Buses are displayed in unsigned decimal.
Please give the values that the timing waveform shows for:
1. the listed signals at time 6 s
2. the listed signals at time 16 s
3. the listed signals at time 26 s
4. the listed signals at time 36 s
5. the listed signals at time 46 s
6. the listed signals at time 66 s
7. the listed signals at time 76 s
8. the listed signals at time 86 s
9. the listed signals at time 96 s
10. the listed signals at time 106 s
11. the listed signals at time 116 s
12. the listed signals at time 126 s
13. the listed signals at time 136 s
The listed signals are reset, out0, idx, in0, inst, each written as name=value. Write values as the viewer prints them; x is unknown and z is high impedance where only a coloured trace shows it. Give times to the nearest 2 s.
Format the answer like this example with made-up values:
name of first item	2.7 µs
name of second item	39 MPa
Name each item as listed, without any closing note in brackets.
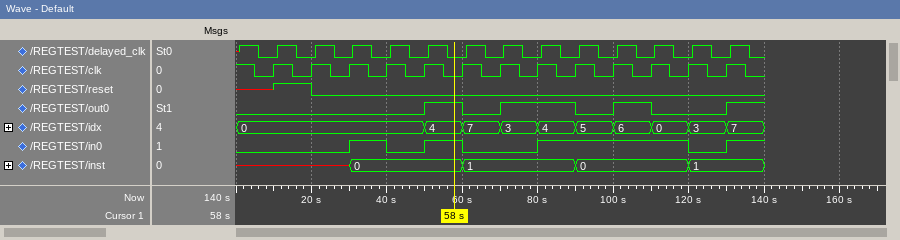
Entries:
the listed signals at time 6 s	reset=x, out0=0, idx=0, in0=0, inst=x
the listed signals at time 16 s	reset=1, out0=0, idx=0, in0=0, inst=x
the listed signals at time 26 s	reset=0, out0=0, idx=0, in0=0, inst=x
the listed signals at time 36 s	reset=0, out0=0, idx=0, in0=1, inst=0
the listed signals at time 46 s	reset=0, out0=0, idx=0, in0=0, inst=0
the listed signals at time 66 s	reset=0, out0=0, idx=7, in0=0, inst=1
the listed signals at time 76 s	reset=0, out0=1, idx=3, in0=0, inst=1
the listed signals at time 86 s	reset=0, out0=1, idx=4, in0=1, inst=1
the listed signals at time 96 s	reset=0, out0=0, idx=5, in0=1, inst=0
the listed signals at time 106 s	reset=0, out0=1, idx=6, in0=1, inst=0
the listed signals at time 116 s	reset=0, out0=0, idx=0, in0=1, inst=0
the listed signals at time 126 s	reset=0, out0=0, idx=3, in0=0, inst=1
the listed signals at time 136 s	reset=0, out0=1, idx=7, in0=1, inst=1
